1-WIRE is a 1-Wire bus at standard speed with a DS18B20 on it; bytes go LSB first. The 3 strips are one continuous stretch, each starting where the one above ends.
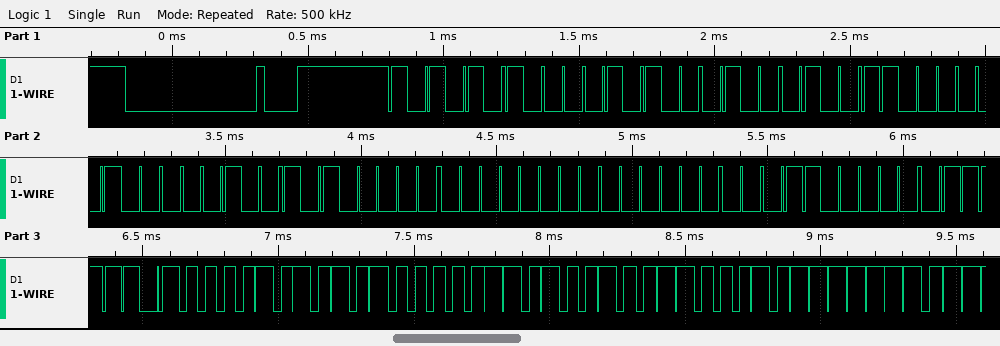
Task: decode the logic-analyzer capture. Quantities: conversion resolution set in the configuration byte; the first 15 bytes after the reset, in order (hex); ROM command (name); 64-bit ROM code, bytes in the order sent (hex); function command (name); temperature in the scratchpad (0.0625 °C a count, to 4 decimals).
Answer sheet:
12 bits
55 28 22 83 20 05 00 00 06 BE 50 05 4B 46 7F
Match ROM
28 22 83 20 05 00 00 06
Read Scratchpad
85.0000 °C
